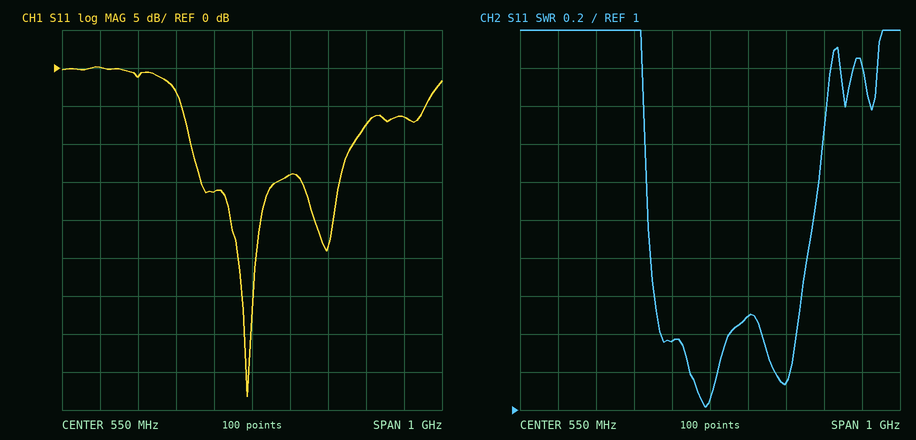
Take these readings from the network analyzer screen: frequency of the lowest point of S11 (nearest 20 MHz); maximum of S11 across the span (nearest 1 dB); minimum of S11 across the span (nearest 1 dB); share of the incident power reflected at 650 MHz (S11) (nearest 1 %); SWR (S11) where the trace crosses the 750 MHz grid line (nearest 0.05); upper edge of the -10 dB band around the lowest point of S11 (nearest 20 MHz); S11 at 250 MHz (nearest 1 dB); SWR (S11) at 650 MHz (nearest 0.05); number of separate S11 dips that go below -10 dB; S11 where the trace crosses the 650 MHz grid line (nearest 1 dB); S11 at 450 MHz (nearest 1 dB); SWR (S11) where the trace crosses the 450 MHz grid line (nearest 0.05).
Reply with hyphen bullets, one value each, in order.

- 540 MHz
- 0 dB
- -43 dB
- 4 %
- 1.15
- 820 MHz
- -1 dB
- 1.50
- 2
- -14 dB
- -16 dB
- 1.35
